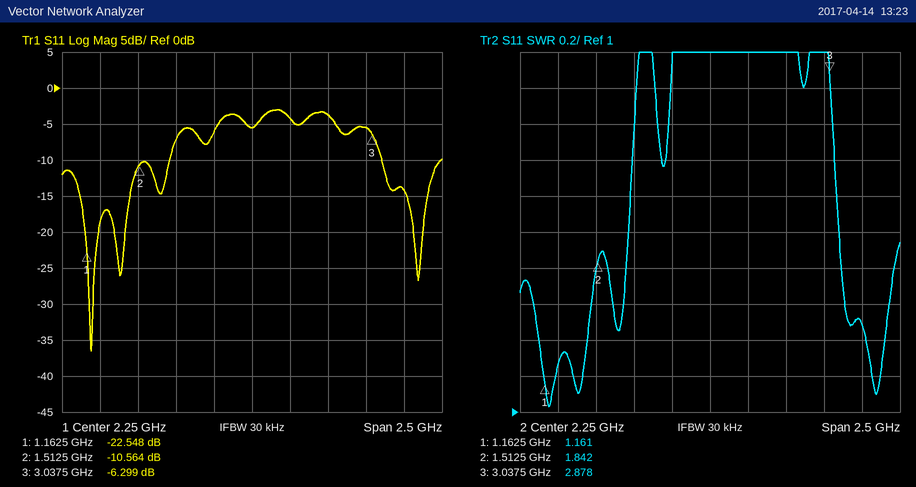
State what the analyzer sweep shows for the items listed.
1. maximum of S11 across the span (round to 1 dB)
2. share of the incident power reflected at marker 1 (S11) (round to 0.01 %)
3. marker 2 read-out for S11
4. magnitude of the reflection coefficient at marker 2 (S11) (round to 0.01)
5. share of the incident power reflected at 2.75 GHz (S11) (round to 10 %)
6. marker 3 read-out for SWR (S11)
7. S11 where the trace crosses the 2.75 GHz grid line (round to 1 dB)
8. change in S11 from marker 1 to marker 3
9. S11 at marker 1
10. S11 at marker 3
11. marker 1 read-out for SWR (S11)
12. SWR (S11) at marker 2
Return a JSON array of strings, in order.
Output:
["-3 dB", "0.56 %", "-10.564 dB", "0.30", "40 %", "2.878", "-4 dB", "16.249 dB", "-22.548 dB", "-6.299 dB", "1.161", "1.842"]
